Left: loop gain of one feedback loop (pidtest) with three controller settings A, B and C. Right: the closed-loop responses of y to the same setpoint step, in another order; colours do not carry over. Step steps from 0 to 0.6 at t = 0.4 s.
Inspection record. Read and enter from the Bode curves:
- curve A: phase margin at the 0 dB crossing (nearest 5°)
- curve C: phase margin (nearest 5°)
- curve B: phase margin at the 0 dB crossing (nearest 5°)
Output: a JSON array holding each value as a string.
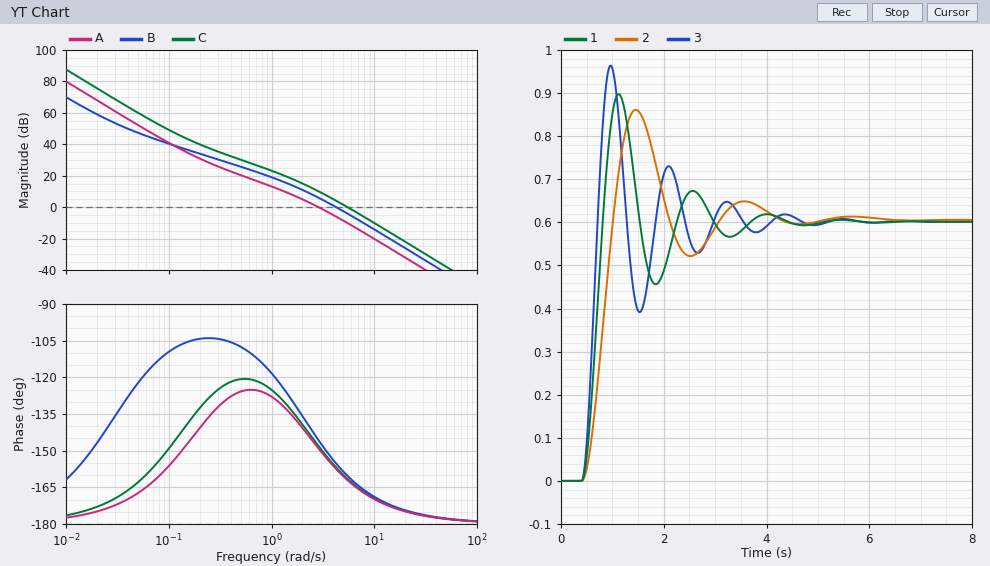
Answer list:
["30°", "20°", "25°"]
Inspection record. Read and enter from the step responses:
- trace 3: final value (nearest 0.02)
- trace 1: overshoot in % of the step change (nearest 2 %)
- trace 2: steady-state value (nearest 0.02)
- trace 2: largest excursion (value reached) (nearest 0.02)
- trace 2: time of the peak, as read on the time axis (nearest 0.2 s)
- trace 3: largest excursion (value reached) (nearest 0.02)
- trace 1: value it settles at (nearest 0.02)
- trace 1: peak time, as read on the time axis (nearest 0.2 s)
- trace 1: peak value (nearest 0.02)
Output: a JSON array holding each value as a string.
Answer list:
["0.60", "50 %", "0.60", "0.86", "1.4 s", "0.96", "0.60", "1.2 s", "0.90"]
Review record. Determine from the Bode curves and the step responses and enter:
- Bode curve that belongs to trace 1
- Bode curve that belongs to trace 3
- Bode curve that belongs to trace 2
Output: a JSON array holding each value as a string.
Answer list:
["B", "C", "A"]
